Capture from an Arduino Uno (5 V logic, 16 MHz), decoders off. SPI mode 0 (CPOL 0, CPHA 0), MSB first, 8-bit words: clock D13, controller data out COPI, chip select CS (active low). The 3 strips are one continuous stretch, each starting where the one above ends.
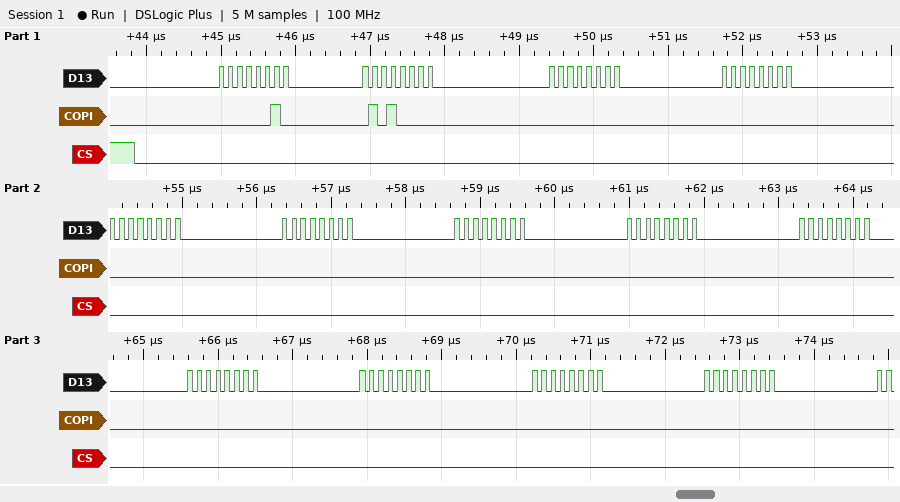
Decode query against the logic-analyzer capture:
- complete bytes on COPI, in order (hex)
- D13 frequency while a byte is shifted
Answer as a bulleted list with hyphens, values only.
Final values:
- 0x02 0x50 0x00 0x00 0x00 0x00 0x00 0x00 0x00 0x00 0x00 0x00 0x00
- 8 MHz
